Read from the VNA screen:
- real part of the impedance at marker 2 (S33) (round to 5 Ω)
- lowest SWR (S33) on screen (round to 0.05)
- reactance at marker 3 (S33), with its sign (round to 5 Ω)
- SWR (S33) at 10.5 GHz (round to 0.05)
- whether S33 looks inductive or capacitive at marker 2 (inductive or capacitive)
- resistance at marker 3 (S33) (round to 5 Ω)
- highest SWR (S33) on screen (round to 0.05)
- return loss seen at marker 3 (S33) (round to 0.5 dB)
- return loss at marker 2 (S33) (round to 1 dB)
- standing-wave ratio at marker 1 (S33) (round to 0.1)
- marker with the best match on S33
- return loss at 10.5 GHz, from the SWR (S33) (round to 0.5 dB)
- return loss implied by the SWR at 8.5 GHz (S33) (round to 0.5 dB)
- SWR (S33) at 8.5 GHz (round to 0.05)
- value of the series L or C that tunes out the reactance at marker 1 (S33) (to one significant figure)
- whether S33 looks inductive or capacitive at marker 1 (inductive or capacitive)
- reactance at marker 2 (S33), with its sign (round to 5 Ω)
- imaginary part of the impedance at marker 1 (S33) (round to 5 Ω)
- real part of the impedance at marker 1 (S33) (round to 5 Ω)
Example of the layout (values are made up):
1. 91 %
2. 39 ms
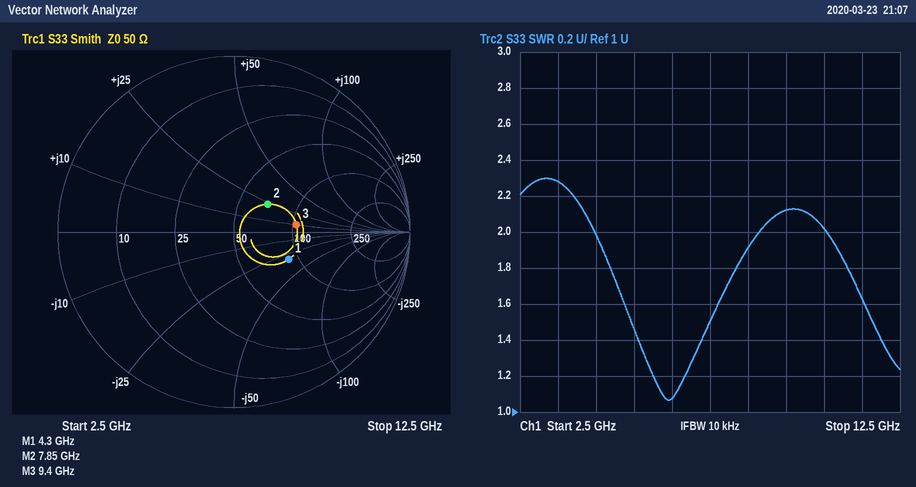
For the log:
1. 70 Ω
2. 1.05
3. +10 Ω
4. 2.00
5. inductive
6. 105 Ω
7. 2.30
8. 9.0 dB
9. 12 dB
10. 2.1
11. marker 2
12. 9.5 dB
13. 10.0 dB
14. 1.90
15. 1 nH
16. capacitive
17. +25 Ω
18. -30 Ω
19. 90 Ω
